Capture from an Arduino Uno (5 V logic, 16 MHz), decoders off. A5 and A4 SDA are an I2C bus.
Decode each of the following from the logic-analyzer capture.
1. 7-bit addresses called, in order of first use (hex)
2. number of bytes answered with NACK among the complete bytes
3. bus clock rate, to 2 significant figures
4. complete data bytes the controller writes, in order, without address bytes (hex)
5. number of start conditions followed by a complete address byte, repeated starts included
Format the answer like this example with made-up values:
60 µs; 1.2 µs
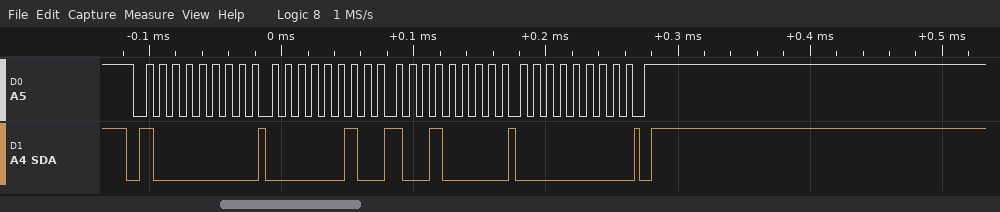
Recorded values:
0x40; 0; 100 kHz; 02 90 00; 1
